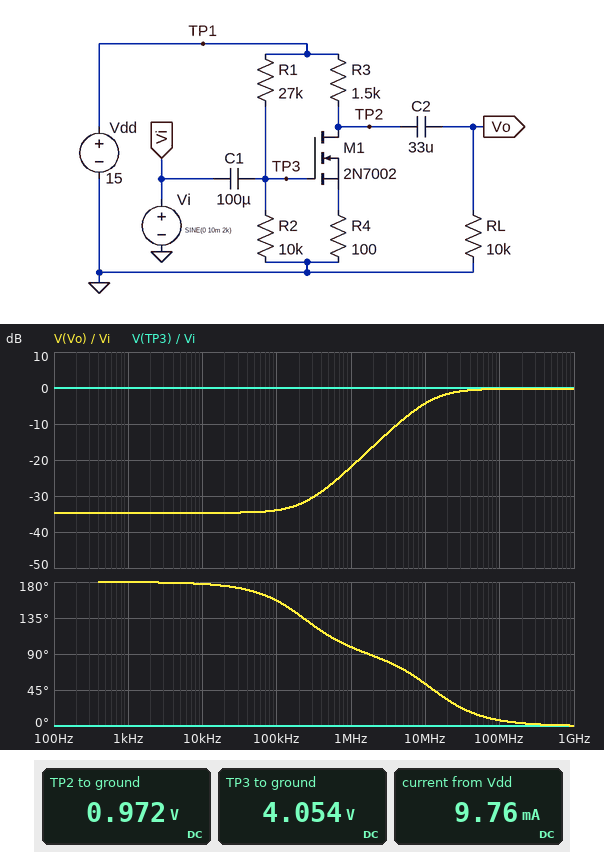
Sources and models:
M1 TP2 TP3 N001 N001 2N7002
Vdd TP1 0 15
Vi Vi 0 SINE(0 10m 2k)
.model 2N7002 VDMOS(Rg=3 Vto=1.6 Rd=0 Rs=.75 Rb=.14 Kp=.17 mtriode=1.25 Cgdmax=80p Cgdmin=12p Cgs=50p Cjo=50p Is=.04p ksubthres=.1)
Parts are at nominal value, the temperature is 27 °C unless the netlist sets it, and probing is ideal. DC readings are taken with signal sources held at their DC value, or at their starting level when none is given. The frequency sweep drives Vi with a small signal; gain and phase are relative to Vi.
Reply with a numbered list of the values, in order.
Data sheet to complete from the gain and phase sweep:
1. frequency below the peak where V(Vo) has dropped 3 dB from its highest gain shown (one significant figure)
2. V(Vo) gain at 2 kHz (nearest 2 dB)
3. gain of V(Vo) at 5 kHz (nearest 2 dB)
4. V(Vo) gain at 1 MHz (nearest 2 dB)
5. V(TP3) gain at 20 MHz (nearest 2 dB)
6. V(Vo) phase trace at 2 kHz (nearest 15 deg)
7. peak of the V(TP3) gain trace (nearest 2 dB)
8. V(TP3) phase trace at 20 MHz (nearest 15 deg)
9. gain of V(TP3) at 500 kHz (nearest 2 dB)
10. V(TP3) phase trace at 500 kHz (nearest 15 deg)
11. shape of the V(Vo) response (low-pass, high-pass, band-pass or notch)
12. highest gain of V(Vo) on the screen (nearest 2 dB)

1. 10 MHz
2. -34 dB
3. -34 dB
4. -22 dB
5. 0 dB
6. 180 deg
7. 0 dB
8. 0 deg
9. 0 dB
10. 0 deg
11. high-pass
12. 0 dB
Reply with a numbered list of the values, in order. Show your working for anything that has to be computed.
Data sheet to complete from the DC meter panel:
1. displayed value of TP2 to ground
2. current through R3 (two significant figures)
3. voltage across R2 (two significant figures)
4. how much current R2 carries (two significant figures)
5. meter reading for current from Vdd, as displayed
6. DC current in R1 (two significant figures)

1. 0.972 V
2. (15 V - 972 mV) / 1.5 kΩ = 9.4 mA
3. 4.054 V = 4.1 V
4. (4.054 V) / 10 kΩ = 410 µA
5. 9.76 mA
6. (15 V - 4.054 V) / 27 kΩ = 410 µA
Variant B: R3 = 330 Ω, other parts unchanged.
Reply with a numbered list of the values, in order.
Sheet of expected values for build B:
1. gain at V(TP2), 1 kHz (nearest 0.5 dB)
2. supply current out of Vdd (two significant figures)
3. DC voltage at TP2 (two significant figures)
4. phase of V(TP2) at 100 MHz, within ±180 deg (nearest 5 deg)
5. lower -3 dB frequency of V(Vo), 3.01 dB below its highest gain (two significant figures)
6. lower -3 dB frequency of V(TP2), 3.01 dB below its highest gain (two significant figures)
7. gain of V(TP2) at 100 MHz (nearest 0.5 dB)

1. 9.0 dB
2. 20 mA
3. 8.5 V
4. 35 deg
5. 550 mHz
6. 210 mHz
7. 2.5 dB
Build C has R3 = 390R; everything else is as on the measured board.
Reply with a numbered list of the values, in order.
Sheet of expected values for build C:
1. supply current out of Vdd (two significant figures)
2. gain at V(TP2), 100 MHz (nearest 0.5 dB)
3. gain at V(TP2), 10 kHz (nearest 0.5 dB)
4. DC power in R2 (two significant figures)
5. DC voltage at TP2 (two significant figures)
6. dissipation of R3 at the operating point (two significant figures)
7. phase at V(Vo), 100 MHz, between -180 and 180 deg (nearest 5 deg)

1. 20 mA
2. 2.5 dB
3. 10.5 dB
4. 1.6 mW
5. 7.4 V
6. 150 mW
7. 30 deg
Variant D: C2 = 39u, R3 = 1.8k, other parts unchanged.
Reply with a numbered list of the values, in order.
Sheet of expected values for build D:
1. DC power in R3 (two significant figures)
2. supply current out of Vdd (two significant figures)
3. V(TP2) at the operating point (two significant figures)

1. 110 mW
2. 8.3 mA
3. 820 mV
